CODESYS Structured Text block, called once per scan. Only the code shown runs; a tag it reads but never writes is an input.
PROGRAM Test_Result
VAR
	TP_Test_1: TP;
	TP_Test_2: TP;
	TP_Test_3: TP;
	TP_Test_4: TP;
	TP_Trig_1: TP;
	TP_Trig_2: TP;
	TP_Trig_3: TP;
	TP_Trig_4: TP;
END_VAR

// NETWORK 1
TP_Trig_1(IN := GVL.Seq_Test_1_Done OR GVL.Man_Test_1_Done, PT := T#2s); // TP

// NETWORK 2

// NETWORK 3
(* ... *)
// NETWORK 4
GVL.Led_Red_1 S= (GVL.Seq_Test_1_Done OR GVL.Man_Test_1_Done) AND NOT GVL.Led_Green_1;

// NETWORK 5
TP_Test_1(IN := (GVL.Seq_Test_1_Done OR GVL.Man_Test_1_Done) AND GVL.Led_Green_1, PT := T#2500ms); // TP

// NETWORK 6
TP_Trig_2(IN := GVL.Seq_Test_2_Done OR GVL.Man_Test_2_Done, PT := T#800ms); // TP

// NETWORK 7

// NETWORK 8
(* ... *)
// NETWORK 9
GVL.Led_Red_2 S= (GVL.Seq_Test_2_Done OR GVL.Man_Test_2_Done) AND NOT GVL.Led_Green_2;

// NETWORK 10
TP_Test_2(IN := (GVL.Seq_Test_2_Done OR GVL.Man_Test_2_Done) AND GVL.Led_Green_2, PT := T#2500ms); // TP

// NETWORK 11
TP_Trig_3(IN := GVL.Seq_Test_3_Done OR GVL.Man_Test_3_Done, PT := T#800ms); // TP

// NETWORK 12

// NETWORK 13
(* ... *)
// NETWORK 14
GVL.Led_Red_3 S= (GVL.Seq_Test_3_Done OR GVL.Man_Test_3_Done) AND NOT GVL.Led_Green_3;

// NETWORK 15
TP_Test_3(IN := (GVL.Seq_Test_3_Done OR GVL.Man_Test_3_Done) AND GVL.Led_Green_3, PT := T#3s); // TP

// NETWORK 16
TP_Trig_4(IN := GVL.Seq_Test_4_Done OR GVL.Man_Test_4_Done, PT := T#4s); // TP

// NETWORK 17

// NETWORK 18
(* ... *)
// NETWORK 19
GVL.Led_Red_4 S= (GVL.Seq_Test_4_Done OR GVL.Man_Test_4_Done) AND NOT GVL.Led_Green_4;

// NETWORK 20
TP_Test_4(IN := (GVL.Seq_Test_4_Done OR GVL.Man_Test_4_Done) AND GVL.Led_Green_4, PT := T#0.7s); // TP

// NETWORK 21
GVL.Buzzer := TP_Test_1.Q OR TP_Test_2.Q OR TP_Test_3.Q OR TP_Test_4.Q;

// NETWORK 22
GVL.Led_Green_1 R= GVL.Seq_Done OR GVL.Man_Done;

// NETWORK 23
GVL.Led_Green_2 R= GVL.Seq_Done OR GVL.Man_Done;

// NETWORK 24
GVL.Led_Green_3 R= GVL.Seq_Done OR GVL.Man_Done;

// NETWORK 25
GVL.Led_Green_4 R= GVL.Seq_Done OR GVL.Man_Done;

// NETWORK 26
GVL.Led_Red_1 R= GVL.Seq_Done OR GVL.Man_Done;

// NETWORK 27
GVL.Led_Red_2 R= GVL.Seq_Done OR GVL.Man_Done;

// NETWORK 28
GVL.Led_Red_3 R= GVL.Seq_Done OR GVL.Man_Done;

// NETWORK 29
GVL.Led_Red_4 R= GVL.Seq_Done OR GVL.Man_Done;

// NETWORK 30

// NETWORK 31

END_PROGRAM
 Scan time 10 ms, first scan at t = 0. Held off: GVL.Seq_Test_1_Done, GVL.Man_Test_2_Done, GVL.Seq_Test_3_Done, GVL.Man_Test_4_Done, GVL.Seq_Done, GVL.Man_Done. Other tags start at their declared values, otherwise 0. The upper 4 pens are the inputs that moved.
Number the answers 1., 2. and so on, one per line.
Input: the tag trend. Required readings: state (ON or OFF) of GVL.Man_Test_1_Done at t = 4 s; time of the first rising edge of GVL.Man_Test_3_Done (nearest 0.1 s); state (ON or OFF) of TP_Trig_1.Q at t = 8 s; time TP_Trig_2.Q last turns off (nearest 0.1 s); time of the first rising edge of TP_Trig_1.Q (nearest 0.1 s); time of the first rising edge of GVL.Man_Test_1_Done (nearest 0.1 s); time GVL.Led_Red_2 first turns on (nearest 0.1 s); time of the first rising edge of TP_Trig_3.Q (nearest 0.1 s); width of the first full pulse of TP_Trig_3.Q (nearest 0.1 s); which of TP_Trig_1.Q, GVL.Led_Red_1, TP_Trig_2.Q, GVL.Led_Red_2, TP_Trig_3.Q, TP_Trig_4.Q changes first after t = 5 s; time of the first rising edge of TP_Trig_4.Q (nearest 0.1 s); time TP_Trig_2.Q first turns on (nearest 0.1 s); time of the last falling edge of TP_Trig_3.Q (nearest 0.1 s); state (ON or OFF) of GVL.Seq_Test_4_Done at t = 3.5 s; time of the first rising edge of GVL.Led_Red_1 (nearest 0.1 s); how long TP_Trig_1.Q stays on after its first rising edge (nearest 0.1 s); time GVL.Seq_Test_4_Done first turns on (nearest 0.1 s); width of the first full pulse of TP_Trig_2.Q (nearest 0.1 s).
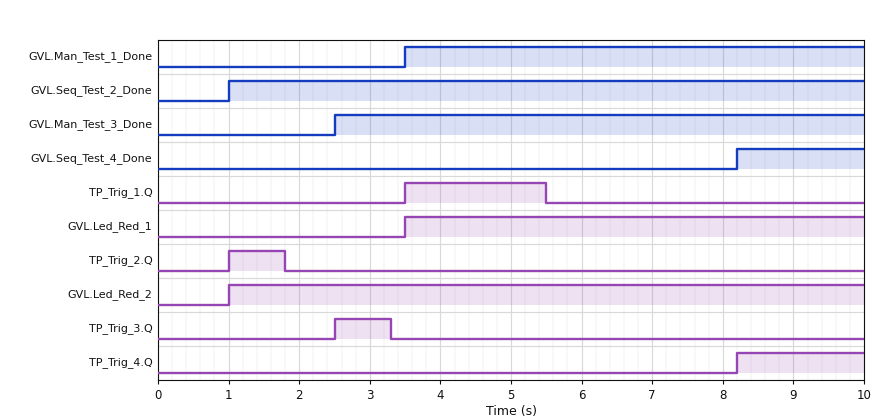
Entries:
1. ON
2. 2.5 s
3. OFF
4. 1.8 s
5. 3.5 s
6. 3.5 s
7. 1.0 s
8. 2.5 s
9. 0.8 s
10. TP_Trig_1.Q
11. 8.2 s
12. 1.0 s
13. 3.3 s
14. OFF
15. 3.5 s
16. 2.0 s
17. 8.2 s
18. 0.8 s
